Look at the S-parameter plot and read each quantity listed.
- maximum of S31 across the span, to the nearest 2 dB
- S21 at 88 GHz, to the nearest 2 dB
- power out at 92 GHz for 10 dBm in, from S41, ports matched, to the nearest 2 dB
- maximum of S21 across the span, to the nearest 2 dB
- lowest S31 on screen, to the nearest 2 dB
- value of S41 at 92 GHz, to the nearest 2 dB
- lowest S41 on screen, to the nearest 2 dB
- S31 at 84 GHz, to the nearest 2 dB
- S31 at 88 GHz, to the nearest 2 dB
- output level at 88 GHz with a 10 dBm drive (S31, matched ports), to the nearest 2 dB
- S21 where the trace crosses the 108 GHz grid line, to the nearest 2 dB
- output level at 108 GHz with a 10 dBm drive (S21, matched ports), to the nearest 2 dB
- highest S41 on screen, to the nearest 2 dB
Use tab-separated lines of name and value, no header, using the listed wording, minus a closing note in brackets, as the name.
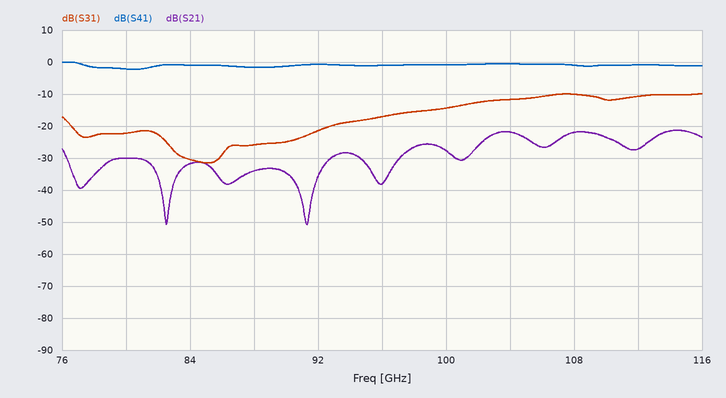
maximum of S31 across the span, to the nearest 2 dB	-10 dB
S21 at 88 GHz, to the nearest 2 dB	-34 dB
power out at 92 GHz for 10 dBm in, from S41, ports matched, to the nearest 2 dB	10 dBm
maximum of S21 across the span, to the nearest 2 dB	-22 dB
lowest S31 on screen, to the nearest 2 dB	-32 dB
value of S41 at 92 GHz, to the nearest 2 dB	0 dB
lowest S41 on screen, to the nearest 2 dB	-2 dB
S31 at 84 GHz, to the nearest 2 dB	-30 dB
S31 at 88 GHz, to the nearest 2 dB	-26 dB
output level at 88 GHz with a 10 dBm drive (S31, matched ports), to the nearest 2 dB	-16 dBm
S21 where the trace crosses the 108 GHz grid line, to the nearest 2 dB	-22 dB
output level at 108 GHz with a 10 dBm drive (S21, matched ports), to the nearest 2 dB	-12 dBm
highest S41 on screen, to the nearest 2 dB	0 dB
